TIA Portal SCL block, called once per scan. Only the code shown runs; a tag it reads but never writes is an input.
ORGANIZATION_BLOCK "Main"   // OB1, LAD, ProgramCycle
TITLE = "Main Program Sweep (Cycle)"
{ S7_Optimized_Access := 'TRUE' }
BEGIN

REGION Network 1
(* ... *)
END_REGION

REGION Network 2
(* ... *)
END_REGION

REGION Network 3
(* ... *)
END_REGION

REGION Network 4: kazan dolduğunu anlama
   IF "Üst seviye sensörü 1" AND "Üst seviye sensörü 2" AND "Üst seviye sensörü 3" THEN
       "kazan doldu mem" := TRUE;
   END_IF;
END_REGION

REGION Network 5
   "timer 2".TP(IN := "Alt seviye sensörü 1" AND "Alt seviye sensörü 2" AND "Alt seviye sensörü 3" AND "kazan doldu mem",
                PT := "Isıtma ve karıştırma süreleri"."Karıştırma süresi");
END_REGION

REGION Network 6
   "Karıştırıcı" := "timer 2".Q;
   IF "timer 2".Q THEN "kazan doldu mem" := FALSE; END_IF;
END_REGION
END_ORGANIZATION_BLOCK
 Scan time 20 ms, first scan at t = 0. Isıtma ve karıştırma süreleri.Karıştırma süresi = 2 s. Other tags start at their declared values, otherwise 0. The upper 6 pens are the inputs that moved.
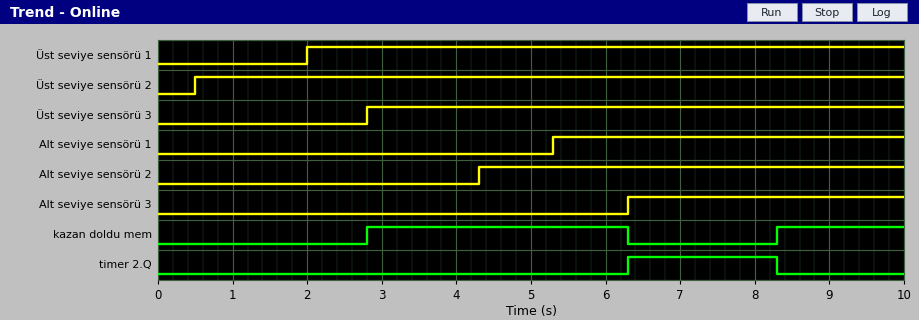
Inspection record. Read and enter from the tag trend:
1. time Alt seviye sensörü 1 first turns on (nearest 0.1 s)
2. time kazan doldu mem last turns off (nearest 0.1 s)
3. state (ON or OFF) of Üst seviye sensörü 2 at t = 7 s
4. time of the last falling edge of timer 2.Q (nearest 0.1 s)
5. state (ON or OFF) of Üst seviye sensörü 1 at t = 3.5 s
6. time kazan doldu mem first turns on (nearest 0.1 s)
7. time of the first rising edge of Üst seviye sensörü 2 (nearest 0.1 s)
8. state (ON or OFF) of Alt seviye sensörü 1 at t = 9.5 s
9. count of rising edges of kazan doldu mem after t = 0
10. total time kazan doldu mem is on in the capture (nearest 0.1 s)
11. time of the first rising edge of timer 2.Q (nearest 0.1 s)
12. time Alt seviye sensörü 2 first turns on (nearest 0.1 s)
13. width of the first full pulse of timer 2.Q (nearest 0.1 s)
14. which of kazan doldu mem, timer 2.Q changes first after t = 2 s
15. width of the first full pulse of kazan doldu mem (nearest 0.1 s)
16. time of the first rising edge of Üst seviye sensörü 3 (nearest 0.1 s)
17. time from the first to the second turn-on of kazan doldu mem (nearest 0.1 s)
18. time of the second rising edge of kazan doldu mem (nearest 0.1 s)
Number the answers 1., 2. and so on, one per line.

1. 5.3 s
2. 6.3 s
3. ON
4. 8.3 s
5. ON
6. 2.8 s
7. 0.5 s
8. ON
9. 2
10. 5.2 s
11. 6.3 s
12. 4.3 s
13. 2.0 s
14. kazan doldu mem
15. 3.5 s
16. 2.8 s
17. 5.5 s
18. 8.3 s
